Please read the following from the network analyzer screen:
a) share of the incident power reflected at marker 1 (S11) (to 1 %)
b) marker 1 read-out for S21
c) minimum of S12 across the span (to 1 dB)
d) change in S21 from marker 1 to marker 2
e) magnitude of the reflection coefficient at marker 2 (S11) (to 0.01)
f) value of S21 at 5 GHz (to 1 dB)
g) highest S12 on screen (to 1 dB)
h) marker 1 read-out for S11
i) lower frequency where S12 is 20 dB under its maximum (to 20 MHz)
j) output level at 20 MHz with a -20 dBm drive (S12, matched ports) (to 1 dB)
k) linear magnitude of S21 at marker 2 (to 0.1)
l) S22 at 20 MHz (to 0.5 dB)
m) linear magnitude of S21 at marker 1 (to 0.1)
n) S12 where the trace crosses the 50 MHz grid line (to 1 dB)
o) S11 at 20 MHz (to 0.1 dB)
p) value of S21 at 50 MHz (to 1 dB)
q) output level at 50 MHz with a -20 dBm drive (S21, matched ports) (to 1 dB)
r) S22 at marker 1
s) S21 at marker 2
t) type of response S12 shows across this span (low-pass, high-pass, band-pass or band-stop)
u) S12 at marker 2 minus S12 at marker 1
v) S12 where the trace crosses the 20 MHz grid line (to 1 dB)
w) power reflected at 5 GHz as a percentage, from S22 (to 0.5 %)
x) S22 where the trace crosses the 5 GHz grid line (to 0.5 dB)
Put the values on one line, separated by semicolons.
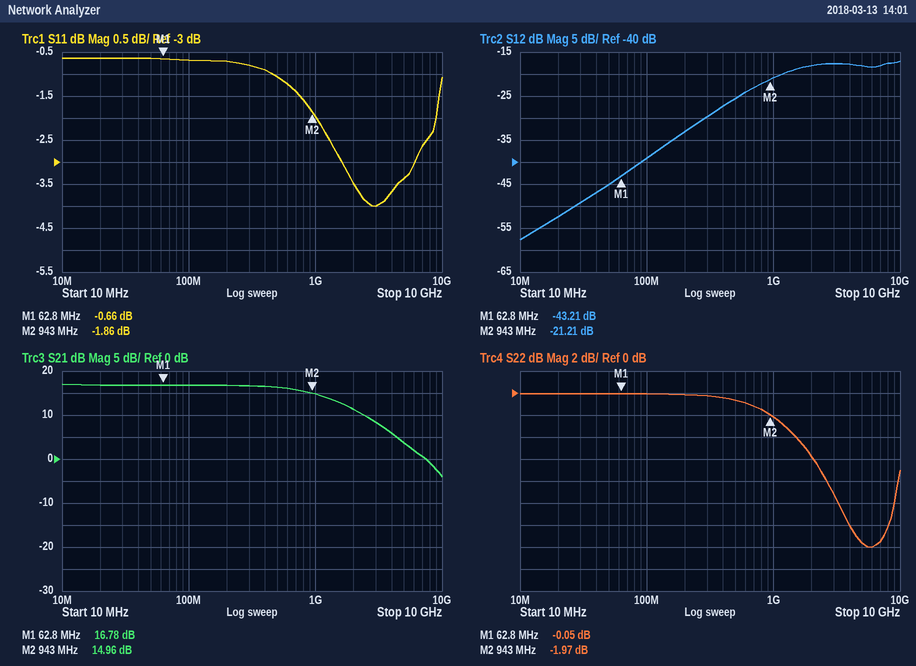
86 %; 16.78 dB; -58 dB; -1.82 dB; 0.81; 4 dB; -17 dB; -0.66 dB; 120 MHz; -72 dBm; 5.6; 0.0 dB; 6.9; -45 dB; -0.6 dB; 17 dB; -3 dBm; -0.05 dB; 14.96 dB; high-pass; 22.00 dB; -52 dB; 4.5 %; -13.5 dB
